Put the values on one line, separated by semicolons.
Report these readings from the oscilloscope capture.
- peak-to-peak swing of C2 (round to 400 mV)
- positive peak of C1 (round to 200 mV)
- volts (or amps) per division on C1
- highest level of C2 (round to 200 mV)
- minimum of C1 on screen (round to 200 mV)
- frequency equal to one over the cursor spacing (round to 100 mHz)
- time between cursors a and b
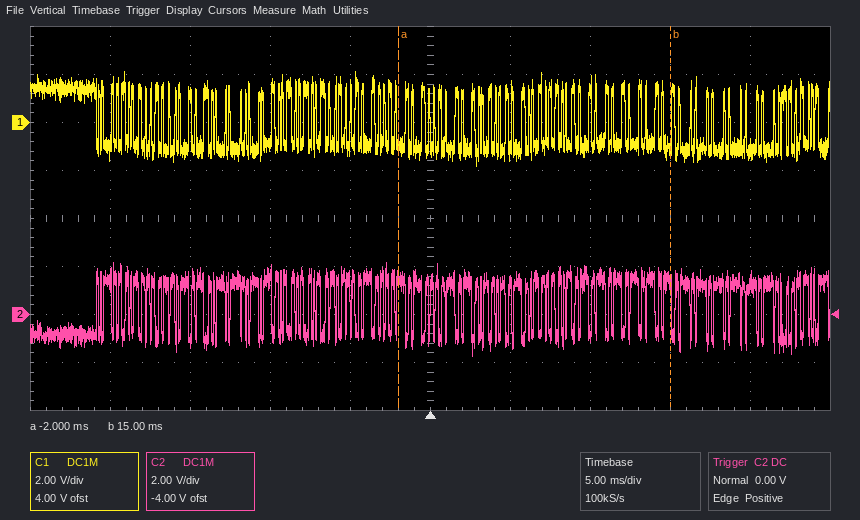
4.0 V; 2.2 V; 2 V; 2.2 V; -1.8 V; 58.8 Hz; 17.0 ms
